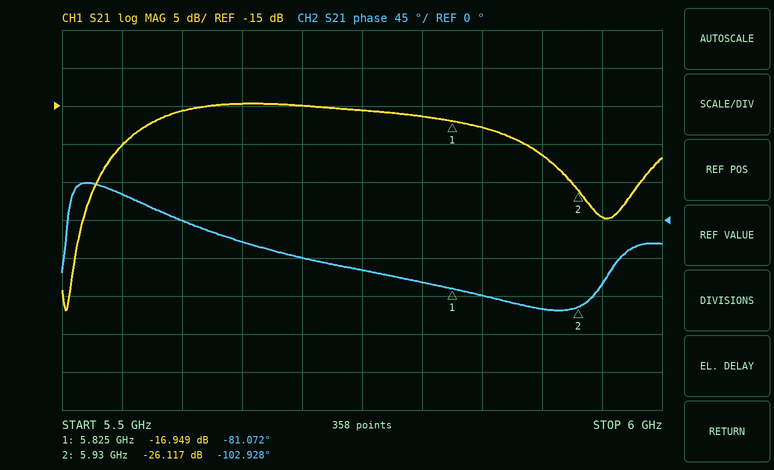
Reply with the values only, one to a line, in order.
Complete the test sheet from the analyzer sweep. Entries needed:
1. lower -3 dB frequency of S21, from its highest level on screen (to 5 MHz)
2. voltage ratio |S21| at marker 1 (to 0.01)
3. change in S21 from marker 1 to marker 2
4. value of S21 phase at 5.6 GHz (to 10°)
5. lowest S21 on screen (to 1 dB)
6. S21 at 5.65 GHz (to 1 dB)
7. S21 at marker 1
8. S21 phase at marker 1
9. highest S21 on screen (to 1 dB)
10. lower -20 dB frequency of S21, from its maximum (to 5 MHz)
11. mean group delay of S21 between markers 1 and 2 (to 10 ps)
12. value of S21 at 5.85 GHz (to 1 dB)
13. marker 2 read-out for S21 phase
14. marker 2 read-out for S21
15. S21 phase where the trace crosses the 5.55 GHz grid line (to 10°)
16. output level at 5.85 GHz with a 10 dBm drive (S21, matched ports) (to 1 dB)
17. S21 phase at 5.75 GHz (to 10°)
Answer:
5.570 GHz
0.14
-9.168 dB
0°
-42 dB
-15 dB
-16.949 dB
-81.072°
-15 dB
5.510 GHz
580 ps
-18 dB
-102.928°
-26.117 dB
30°
-8 dBm
-60°
